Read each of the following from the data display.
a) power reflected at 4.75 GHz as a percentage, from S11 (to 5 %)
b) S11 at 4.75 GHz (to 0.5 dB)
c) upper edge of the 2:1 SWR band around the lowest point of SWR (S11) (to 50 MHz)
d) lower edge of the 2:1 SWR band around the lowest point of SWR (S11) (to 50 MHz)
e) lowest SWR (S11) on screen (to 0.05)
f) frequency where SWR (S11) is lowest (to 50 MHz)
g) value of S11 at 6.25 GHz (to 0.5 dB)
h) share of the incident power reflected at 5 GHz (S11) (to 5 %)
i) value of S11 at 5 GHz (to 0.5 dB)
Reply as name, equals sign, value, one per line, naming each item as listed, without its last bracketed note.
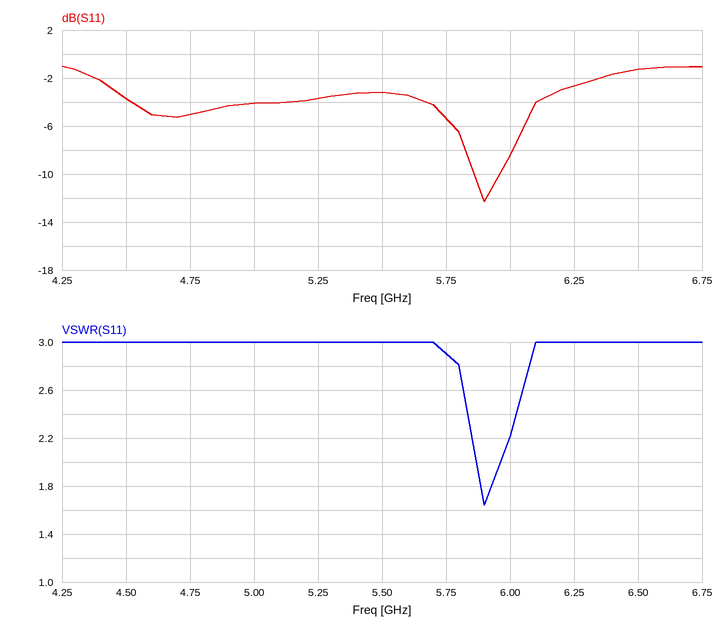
power reflected at 4.75 GHz as a percentage, from S11 = 30 %
S11 at 4.75 GHz = -5.0 dB
upper edge of the 2:1 SWR band around the lowest point of SWR (S11) = 5.95 GHz
lower edge of the 2:1 SWR band around the lowest point of SWR (S11) = 5.85 GHz
lowest SWR (S11) on screen = 1.65
frequency where SWR (S11) is lowest = 5.90 GHz
value of S11 at 6.25 GHz = -2.5 dB
share of the incident power reflected at 5 GHz (S11) = 40 %
value of S11 at 5 GHz = -4.0 dB
